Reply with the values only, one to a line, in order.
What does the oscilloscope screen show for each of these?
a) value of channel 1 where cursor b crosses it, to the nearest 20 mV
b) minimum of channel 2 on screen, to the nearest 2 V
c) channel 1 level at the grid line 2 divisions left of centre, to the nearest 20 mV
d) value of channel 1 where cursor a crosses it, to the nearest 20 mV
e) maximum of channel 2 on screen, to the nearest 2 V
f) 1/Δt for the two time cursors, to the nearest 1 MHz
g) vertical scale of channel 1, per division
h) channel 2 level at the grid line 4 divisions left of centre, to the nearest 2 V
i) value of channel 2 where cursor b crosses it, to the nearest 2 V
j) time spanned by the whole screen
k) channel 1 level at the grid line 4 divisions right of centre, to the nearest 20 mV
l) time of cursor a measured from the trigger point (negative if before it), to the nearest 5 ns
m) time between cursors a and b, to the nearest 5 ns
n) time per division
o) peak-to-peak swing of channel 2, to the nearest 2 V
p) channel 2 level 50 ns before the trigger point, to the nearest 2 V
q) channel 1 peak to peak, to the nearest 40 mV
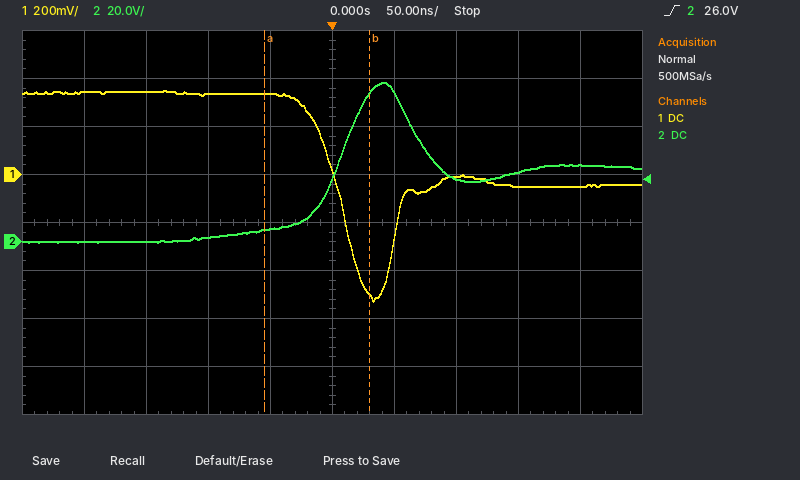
-500 mV
0 V
340 mV
340 mV
66 V
12 MHz
200 mV
0 V
62 V
500 ns
-40 mV
-55 ns
85 ns
50 ns
66 V
6 V
880 mV
